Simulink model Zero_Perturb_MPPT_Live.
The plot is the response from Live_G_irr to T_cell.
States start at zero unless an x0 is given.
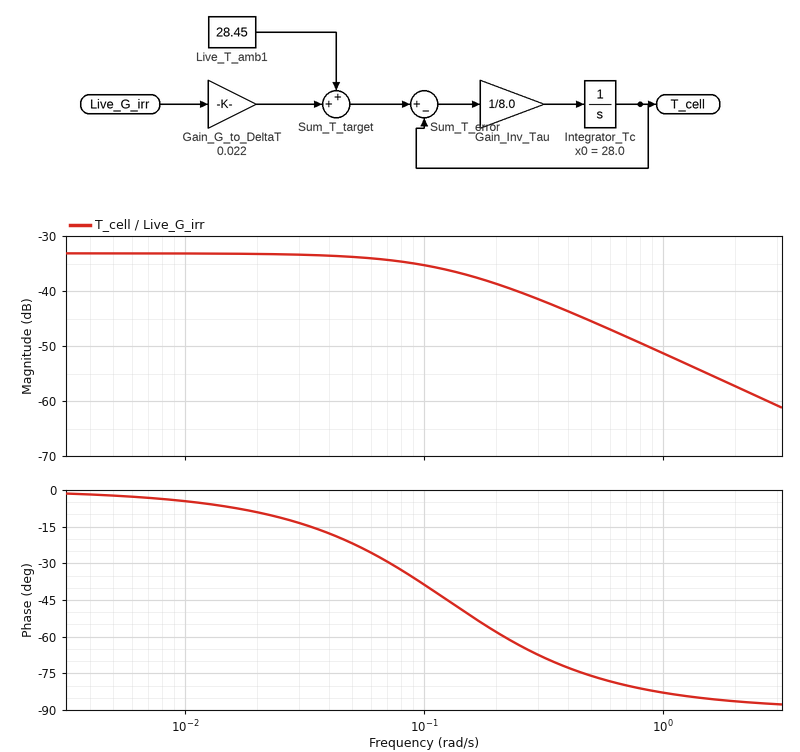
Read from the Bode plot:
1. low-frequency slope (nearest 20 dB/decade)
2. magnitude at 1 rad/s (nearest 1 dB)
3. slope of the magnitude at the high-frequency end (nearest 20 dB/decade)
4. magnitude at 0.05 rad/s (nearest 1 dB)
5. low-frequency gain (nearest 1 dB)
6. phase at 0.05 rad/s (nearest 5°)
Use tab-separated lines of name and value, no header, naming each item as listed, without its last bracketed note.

low-frequency slope	0 dB/decade
magnitude at 1 rad/s	-51 dB
slope of the magnitude at the high-frequency end	-20 dB/decade
magnitude at 0.05 rad/s	-34 dB
low-frequency gain	-33 dB
phase at 0.05 rad/s	-20°
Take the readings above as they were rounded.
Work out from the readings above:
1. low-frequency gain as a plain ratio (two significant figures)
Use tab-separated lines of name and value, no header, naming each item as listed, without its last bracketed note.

low-frequency gain as a plain ratio	0.022
